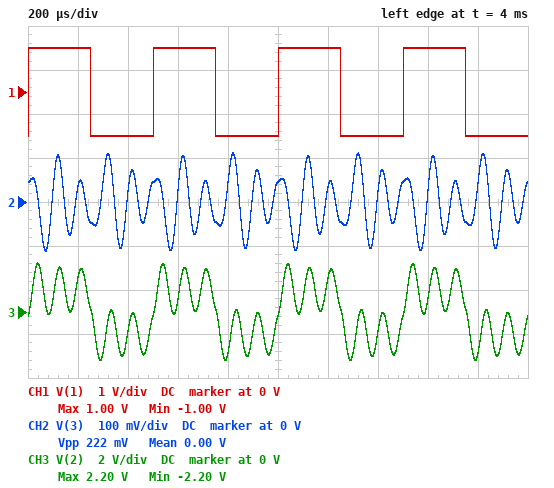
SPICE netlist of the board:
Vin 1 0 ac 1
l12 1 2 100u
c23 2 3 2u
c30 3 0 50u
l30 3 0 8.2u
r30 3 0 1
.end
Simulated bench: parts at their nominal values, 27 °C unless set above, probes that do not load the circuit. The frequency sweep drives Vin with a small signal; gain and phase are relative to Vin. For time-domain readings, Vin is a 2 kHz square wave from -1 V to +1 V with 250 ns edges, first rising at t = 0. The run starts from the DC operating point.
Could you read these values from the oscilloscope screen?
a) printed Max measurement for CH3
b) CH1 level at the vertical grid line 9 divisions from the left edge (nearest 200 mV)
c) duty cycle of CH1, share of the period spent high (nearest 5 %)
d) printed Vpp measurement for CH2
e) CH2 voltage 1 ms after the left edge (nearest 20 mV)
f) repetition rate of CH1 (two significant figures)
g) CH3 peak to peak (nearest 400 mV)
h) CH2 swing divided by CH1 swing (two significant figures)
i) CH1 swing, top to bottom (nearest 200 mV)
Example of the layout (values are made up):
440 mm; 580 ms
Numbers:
2.20 V; -1.0 V; 50 %; 222 mV; 40 mV; 2.0 kHz; 4.4 V; 0.11; 2.0 V
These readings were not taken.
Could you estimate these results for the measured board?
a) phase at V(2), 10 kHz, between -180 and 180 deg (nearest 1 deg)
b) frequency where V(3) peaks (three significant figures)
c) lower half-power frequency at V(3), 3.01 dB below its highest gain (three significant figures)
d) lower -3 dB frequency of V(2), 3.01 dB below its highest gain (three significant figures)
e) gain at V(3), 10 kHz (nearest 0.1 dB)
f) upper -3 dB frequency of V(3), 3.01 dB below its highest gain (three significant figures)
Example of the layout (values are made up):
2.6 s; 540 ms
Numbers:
-8 deg; 11.6 kHz; 11.4 kHz; 11.4 kHz; -10.7 dB; 11.7 kHz
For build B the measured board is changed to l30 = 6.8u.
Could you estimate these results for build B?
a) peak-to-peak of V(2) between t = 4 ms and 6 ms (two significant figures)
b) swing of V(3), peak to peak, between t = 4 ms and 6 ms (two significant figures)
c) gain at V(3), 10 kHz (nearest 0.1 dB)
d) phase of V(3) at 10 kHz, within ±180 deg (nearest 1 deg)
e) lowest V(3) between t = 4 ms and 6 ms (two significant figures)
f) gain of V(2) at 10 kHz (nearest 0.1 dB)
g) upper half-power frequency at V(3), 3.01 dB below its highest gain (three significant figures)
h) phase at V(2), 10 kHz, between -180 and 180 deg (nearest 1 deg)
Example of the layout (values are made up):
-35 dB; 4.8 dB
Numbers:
4.4 V; 240 mV; -9.2 dB; 36 deg; -120 mV; 11.5 dB; 11.8 kHz; -12 deg
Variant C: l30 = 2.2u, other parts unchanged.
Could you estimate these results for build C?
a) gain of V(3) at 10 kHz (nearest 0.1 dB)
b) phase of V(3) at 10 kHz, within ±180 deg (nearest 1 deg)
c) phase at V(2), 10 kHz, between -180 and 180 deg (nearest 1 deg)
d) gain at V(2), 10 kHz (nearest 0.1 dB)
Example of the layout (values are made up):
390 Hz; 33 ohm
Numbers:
-15.7 dB; 164 deg; -2 deg; 14.6 dB
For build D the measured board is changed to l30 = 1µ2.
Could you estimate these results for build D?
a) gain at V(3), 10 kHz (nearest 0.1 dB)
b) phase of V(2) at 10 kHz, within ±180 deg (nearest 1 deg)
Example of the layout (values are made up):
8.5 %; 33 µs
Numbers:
-24.1 dB; 0 deg
